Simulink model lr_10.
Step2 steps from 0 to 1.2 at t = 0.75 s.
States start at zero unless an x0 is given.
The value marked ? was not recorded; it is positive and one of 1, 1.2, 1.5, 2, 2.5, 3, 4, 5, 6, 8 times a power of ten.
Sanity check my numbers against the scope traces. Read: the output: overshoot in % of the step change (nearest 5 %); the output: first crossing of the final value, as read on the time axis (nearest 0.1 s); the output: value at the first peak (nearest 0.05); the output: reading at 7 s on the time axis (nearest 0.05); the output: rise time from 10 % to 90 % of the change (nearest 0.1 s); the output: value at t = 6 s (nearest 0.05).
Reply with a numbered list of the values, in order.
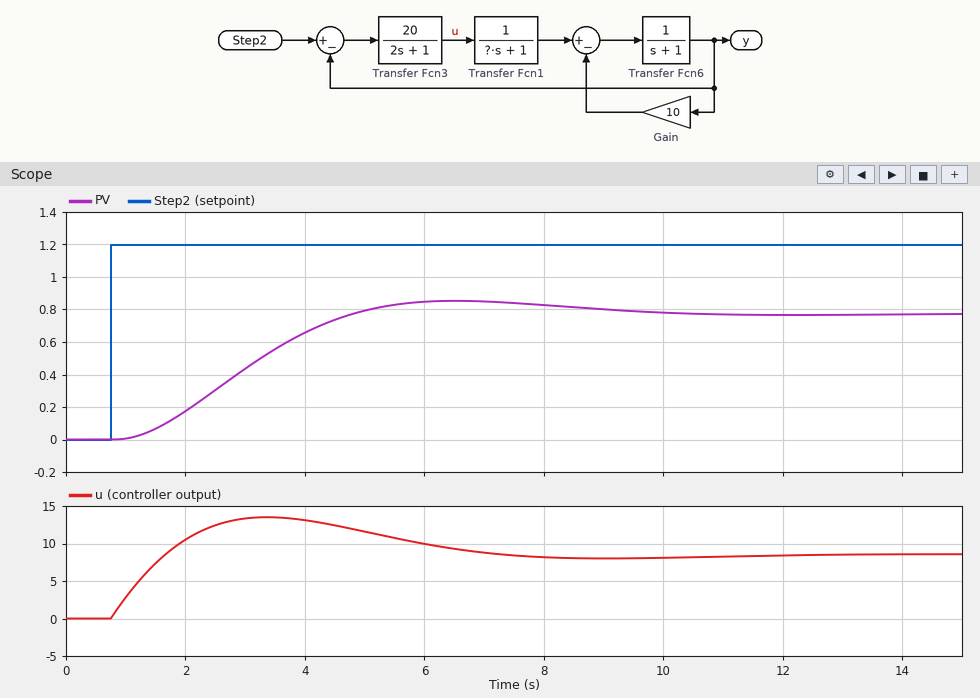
1. 10 %
2. 4.8 s
3. 0.85
4. 0.85
5. 2.7 s
6. 0.85
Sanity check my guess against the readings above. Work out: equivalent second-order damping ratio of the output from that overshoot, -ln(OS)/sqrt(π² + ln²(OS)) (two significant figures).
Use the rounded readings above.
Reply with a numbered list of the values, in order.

1. 0.59
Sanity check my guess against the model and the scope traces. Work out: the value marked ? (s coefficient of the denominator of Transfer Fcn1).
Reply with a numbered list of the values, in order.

1. 3
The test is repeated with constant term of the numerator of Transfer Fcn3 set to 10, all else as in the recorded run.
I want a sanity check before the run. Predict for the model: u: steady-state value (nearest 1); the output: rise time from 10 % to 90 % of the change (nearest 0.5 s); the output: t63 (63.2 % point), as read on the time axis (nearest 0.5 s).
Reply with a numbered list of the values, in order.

1. 6
2. 4.0 s
3. 4.0 s
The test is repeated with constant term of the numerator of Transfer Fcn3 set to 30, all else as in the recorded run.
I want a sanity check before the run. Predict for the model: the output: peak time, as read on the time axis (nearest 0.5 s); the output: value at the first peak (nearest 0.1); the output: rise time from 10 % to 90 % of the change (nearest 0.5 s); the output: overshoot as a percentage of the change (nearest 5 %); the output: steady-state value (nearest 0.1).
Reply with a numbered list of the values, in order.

1. 5.5 s
2. 1.0
3. 2.0 s
4. 15 %
5. 0.9
